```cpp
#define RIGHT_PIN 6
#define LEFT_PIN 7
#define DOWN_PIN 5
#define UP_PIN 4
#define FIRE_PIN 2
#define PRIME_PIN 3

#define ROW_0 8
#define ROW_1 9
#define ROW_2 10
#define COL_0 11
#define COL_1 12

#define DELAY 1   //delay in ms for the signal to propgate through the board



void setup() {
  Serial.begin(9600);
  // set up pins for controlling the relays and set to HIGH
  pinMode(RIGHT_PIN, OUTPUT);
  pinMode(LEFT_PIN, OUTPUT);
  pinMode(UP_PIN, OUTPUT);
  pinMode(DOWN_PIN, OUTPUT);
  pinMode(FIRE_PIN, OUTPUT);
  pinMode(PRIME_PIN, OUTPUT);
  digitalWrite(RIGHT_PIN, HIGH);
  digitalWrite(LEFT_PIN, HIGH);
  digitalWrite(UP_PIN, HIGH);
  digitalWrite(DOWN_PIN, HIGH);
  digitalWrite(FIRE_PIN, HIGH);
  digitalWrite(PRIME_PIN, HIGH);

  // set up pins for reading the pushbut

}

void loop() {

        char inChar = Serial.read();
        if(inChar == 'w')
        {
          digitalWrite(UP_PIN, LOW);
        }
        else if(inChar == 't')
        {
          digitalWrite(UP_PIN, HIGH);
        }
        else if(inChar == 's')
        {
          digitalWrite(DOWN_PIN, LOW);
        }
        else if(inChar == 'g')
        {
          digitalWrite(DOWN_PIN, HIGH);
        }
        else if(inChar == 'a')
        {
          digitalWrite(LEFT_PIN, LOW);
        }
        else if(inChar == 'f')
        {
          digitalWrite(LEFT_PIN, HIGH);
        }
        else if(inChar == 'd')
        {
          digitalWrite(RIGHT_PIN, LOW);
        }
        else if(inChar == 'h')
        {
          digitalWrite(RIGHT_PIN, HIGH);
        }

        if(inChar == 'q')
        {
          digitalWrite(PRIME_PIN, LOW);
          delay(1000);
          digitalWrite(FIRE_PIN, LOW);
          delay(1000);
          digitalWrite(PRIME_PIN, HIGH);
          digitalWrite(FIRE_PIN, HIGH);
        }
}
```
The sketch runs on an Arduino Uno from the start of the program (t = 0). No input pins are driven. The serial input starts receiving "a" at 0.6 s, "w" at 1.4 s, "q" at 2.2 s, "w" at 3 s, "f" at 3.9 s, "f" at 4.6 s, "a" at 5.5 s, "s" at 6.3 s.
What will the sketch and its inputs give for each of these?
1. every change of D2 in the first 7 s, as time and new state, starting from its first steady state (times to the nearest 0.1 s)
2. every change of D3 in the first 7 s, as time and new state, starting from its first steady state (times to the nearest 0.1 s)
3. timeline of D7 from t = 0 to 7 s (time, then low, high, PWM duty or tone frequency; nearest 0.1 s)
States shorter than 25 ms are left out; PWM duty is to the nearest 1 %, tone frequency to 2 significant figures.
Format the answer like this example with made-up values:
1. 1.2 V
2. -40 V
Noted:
1. 0 s high; 3.2 s low; 4.2 s high
2. 0 s high; 2.2 s low; 4.2 s high
3. 0 s high; 0.6 s low; 4.2 s high; 5.5 s low
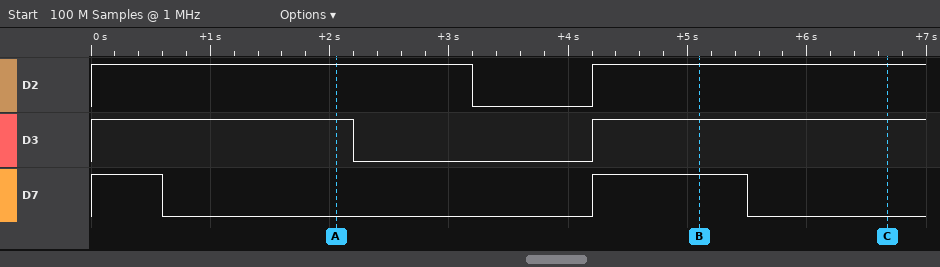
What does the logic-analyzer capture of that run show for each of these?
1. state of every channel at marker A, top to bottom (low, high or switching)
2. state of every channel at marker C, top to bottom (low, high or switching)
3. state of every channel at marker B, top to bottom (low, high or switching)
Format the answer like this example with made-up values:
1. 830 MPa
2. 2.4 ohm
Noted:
1. D2 high, D3 high, D7 low
2. D2 high, D3 high, D7 low
3. D2 high, D3 high, D7 high
